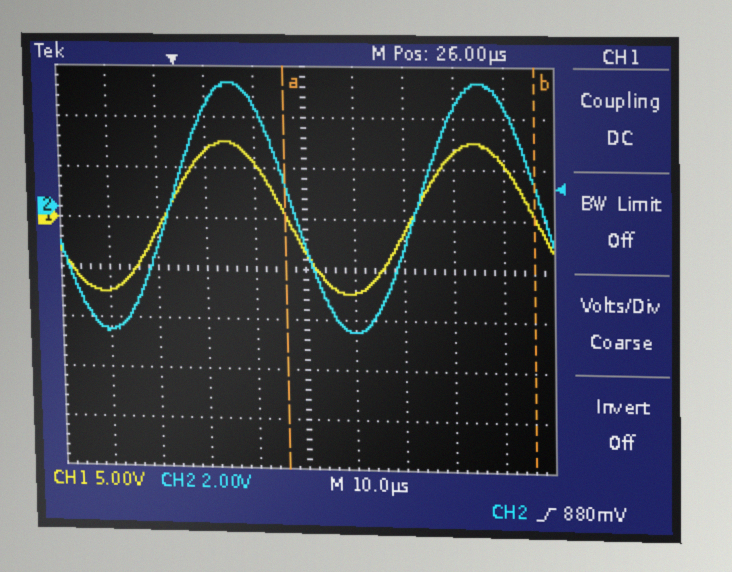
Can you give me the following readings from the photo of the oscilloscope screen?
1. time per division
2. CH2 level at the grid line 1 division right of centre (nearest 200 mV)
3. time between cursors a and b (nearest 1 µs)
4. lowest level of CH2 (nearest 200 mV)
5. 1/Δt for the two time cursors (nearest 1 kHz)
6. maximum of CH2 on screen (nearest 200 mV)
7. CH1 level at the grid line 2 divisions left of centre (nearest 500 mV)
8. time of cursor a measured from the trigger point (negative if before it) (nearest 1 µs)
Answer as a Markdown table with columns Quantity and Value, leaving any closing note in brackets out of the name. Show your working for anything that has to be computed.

| Quantity | Value |
|---|---|
| time per division | 10 µs |
| CH2 level at the grid line 1 division right of centre | -4.8 V |
| time between cursors a and b | 50 µs |
| lowest level of CH2 | -5.0 V |
| 1/Δt for the two time cursors | 1 / 50 µs ≈ 20 kHz |
| maximum of CH2 on screen | 5.0 V |
| CH1 level at the grid line 2 divisions left of centre | 6.5 V |
| time of cursor a measured from the trigger point (negative if before it) | +22 µs |
